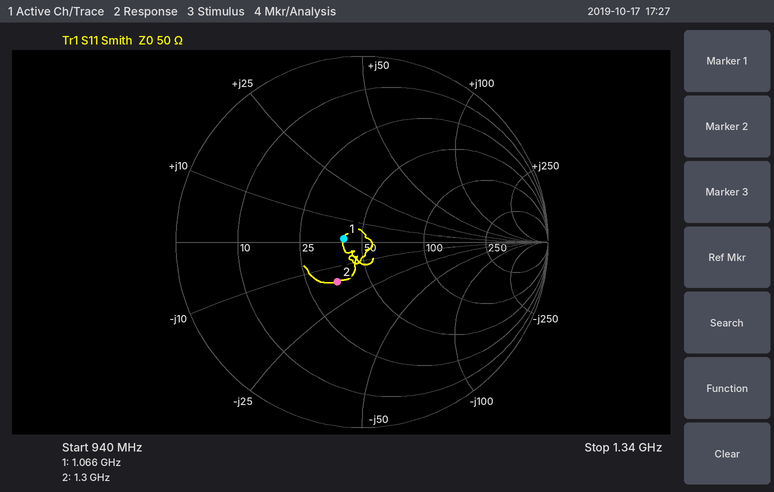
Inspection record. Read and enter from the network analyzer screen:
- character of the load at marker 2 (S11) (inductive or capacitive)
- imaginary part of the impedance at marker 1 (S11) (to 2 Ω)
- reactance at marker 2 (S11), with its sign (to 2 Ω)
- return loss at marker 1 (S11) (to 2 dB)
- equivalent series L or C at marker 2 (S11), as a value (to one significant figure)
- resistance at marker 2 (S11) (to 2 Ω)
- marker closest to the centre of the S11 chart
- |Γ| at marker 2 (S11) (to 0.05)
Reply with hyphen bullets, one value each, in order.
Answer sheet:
- capacitive
- +2 Ω
- -16 Ω
- 20 dB
- 8 pF
- 36 Ω
- marker 1
- 0.25
